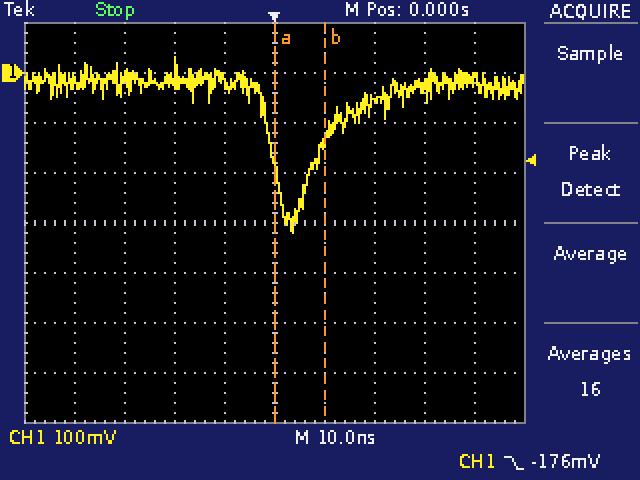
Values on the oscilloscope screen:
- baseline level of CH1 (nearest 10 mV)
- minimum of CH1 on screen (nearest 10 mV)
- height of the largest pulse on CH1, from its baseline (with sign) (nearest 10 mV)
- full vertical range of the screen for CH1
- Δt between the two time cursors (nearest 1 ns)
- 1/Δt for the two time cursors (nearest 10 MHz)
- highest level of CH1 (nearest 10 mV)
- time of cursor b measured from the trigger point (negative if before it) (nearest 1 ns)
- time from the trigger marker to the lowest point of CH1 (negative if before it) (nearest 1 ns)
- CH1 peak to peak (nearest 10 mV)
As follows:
-20 mV
-320 mV
-300 mV
800 mV
10 ns
100 MHz
30 mV
+10 ns
+4 ns
350 mV
